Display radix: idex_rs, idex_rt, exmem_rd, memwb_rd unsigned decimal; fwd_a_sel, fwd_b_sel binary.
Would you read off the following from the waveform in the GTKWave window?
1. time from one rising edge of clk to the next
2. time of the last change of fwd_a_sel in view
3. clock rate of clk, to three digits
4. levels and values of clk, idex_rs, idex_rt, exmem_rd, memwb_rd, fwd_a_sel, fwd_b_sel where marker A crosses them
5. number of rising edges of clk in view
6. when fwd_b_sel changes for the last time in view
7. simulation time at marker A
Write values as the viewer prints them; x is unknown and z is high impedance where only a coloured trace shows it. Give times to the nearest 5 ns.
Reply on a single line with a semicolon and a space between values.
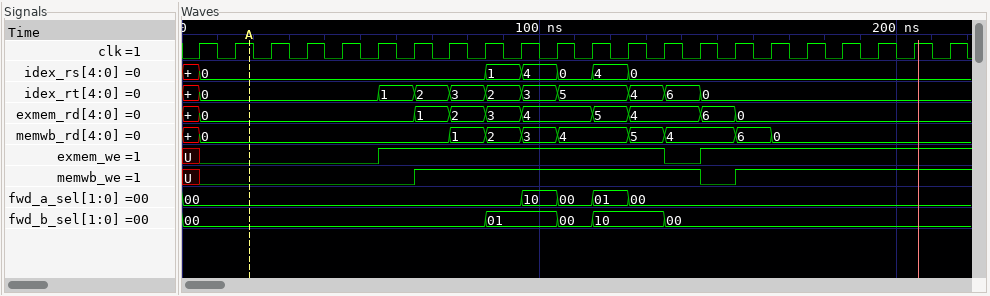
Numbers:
10 ns; 125 ns; 100 MHz; clk=1, idex_rs=0, idex_rt=0, exmem_rd=0, memwb_rd=0, fwd_a_sel=00, fwd_b_sel=00; 22; 135 ns; 20 ns
